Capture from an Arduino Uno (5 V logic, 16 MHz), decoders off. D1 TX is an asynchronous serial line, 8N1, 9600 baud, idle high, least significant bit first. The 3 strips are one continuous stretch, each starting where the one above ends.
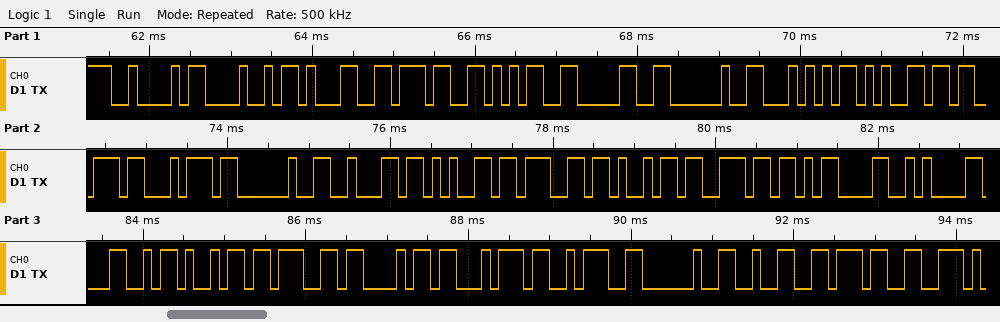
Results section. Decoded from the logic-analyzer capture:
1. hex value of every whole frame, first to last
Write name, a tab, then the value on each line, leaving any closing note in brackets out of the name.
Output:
hex value of every whole frame, first to last	0x42 0x48 0x31 0x37 0x35 0x30 0x20 0x54 0x65 0x73 0x74 0x20 0x62 0x65 0x67 0x69 0x6E 0x0D 0x0A 0x4C 0x69 0x67 0x68 0x74 0x3A 0x20 0x32 0x37
